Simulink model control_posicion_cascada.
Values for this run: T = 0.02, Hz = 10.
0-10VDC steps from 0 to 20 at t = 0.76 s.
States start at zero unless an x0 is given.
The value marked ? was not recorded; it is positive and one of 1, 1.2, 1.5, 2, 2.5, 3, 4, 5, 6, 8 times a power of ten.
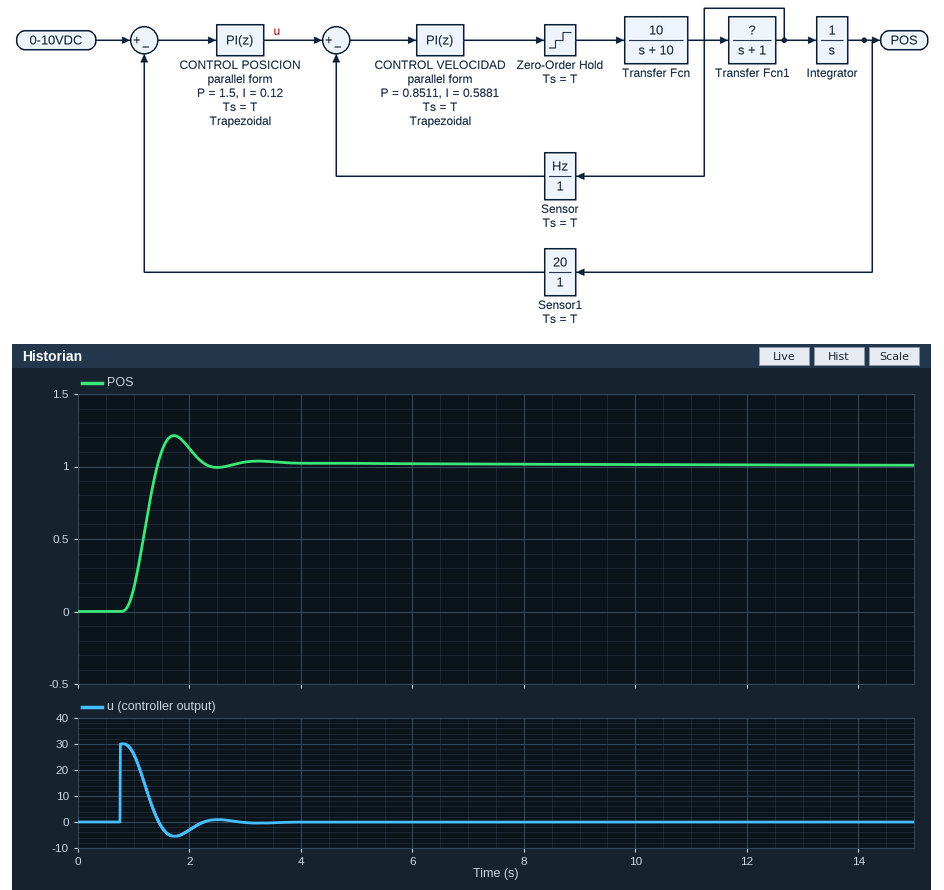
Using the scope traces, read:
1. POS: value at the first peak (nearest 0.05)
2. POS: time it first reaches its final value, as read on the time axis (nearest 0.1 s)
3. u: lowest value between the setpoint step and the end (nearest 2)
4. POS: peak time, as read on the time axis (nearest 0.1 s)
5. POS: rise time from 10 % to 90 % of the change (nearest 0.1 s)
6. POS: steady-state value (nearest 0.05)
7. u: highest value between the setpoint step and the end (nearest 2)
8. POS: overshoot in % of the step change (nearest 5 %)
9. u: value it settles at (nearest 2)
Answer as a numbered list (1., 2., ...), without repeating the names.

1. 1.20
2. 1.4 s
3. -6
4. 1.7 s
5. 0.4 s
6. 1.00
7. 30
8. 20 %
9. 0
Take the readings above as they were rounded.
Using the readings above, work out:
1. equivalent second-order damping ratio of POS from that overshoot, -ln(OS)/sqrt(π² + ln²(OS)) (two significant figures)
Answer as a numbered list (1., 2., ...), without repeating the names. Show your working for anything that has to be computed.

1. ln(0.2) = -1.609; 1.609 / sqrt(9.870 + 2.590) = 0.46
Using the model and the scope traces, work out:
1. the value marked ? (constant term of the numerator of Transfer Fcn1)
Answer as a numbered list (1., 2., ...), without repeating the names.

1. 0.5
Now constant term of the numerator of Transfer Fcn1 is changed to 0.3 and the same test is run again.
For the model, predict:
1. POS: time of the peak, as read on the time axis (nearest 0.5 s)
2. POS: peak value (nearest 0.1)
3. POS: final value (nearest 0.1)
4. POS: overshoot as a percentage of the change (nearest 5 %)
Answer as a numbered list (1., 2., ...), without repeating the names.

1. 2.0 s
2. 1.3
3. 1.0
4. 35 %
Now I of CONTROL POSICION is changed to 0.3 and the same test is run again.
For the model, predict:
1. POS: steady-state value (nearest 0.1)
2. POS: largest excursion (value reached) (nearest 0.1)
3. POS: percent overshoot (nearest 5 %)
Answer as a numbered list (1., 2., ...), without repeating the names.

1. 1.0
2. 1.3
3. 25 %
